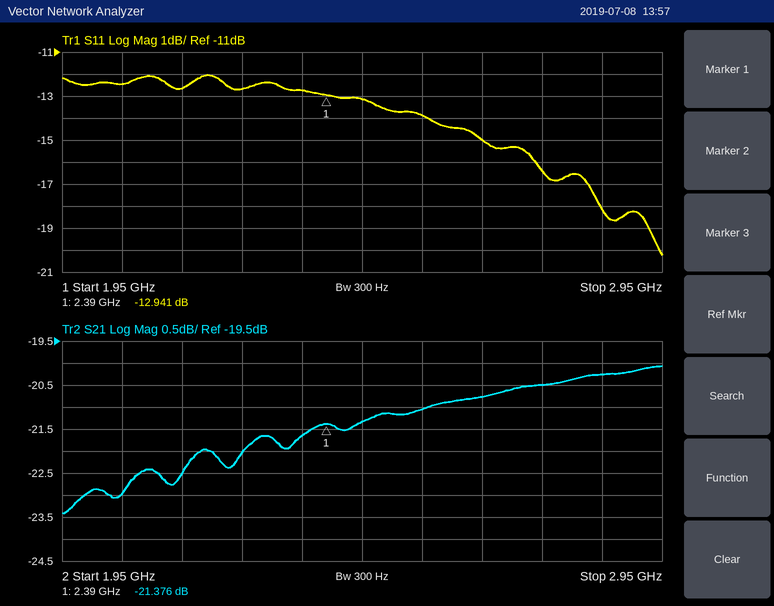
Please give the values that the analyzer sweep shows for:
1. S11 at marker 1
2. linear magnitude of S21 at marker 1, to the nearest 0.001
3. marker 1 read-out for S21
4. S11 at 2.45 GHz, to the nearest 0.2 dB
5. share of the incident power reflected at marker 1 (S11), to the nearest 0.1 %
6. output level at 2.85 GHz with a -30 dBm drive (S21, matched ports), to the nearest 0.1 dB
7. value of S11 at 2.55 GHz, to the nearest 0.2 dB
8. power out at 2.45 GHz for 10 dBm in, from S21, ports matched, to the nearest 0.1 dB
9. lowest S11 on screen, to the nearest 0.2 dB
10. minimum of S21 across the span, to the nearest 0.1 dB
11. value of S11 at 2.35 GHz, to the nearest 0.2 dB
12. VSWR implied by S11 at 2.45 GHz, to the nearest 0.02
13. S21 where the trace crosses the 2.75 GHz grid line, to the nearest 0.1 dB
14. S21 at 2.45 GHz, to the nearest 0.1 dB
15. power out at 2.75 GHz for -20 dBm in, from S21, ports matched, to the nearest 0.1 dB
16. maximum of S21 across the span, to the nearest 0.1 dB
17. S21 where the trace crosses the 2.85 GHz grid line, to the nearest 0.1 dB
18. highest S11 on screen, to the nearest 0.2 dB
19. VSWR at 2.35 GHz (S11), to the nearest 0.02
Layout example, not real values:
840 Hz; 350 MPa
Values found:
-12.941 dB; 0.085; -21.376 dB; -13.2 dB; 5.1 %; -50.3 dBm; -13.8 dB; -11.3 dBm; -20.2 dB; -23.4 dB; -12.8 dB; 1.56; -20.5 dB; -21.3 dB; -40.5 dBm; -20.1 dB; -20.3 dB; -12.0 dB; 1.60
